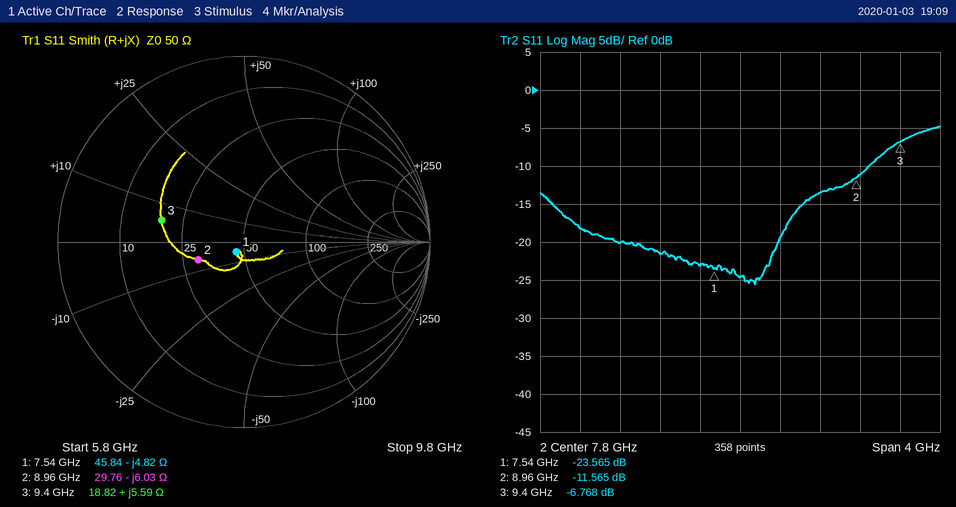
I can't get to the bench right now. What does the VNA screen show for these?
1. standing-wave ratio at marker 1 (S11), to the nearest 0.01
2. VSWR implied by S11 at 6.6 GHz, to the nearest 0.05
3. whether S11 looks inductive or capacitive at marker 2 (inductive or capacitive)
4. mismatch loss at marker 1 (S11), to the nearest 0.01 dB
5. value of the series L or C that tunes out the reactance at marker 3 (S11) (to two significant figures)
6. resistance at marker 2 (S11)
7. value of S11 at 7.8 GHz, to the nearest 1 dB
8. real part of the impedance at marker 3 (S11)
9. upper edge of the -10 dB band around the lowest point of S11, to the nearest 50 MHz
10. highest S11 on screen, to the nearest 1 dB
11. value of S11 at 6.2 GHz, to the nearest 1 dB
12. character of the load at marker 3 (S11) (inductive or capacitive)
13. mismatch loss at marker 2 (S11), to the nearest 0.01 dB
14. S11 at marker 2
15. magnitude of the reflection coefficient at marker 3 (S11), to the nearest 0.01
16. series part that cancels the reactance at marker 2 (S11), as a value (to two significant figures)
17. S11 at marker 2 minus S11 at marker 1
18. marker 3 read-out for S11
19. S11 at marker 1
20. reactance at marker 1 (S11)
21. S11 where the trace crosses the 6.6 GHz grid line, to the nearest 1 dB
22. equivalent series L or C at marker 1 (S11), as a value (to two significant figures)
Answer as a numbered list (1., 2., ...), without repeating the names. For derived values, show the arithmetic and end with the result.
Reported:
1. 1.14
2. |Γ| = 10^(-20/20) = 0.1000; VSWR = (1 + 0.1000)/(1 − 0.1000) ≈ 1.22, so 1.20 to the nearest 0.05
3. capacitive
4. −10 log10(1 − 10^(-23.565/10)) ≈ 0.02 dB
5. C = 1/(2π × 9.4 GHz × 5.59 Ω) ≈ 3.0 pF
6. 29.76 Ω
7. -25 dB
8. 18.82 Ω
9. 9.10 GHz
10. -5 dB
11. -18 dB
12. inductive
13. −10 log10(1 − 10^(-11.565/10)) ≈ 0.31 dB
14. -11.565 dB
15. 0.46
16. L = 6.03 Ω/(2π × 8.96 GHz) ≈ 107 pH, so 110 pH to two significant figures
17. -11.565 − (-23.565) = 12.000 dB
18. -6.768 dB
19. -23.565 dB
20. -4.82 Ω
21. -20 dB
22. C = 1/(2π × 7.54 GHz × 4.82 Ω) ≈ 4.4 pF
